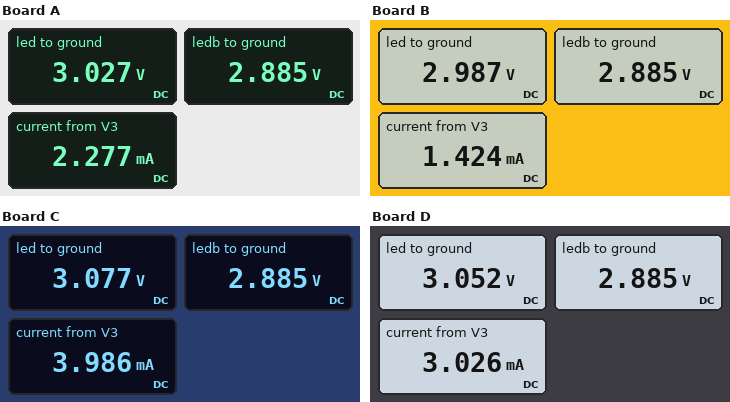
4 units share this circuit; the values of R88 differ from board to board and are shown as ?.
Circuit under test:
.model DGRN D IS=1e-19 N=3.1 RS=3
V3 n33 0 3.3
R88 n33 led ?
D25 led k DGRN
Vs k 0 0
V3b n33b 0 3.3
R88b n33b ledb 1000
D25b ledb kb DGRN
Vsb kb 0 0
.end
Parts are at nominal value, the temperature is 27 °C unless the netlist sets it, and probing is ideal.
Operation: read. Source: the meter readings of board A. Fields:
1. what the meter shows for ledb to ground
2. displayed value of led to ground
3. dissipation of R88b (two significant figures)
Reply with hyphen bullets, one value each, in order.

- 2.885 V
- 3.027 V
- 170 µW
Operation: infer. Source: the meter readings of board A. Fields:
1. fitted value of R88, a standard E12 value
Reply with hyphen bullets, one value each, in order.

- 120 Ω
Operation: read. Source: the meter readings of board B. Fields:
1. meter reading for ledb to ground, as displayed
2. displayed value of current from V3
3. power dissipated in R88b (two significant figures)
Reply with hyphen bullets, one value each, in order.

- 2.885 V
- 1.424 mA
- 170 µW
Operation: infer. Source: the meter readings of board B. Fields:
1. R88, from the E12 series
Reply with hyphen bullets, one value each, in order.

- 220 Ω
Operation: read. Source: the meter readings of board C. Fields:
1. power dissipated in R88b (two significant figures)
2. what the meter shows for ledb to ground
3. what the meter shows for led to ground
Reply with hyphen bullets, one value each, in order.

- 170 µW
- 2.885 V
- 3.077 V
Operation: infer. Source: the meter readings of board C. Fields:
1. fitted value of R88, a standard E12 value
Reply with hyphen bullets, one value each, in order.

- 56 Ω
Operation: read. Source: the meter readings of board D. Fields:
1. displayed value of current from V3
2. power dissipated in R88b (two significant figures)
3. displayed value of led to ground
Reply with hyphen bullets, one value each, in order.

- 3.026 mA
- 170 µW
- 3.052 V
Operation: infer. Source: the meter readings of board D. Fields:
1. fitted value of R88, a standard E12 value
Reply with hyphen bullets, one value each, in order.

- 82 Ω
